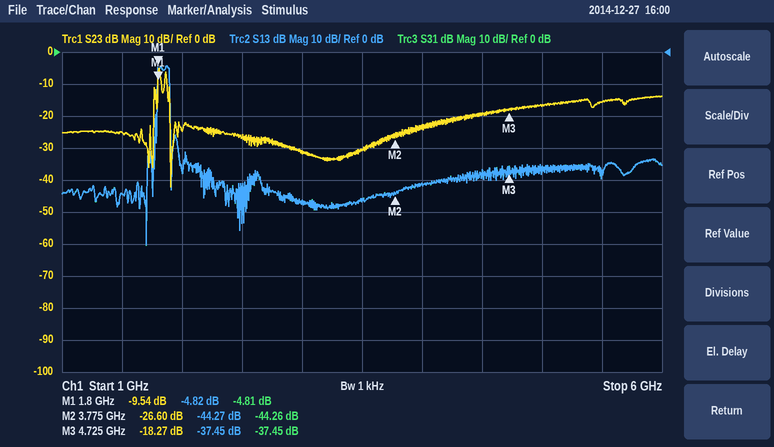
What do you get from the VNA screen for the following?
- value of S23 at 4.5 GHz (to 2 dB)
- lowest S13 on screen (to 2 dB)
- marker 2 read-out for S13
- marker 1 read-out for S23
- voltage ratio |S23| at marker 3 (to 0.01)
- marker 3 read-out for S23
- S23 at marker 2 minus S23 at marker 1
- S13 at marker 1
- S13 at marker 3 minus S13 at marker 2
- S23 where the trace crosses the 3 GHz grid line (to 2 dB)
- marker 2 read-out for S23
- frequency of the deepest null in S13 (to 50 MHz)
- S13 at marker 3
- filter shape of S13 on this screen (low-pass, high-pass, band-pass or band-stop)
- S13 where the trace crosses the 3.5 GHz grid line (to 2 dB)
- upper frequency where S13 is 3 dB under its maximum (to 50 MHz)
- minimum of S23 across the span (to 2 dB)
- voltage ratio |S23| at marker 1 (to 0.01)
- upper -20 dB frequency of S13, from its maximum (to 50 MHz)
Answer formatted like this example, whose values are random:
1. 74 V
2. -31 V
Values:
1. -20 dB
2. -60 dB
3. -44.27 dB
4. -9.54 dB
5. 0.12
6. -18.27 dB
7. -17.06 dB
8. -4.82 dB
9. 6.82 dB
10. -32 dB
11. -26.60 dB
12. 1.70 GHz
13. -37.45 dB
14. band-pass
15. -46 dB
16. 1.90 GHz
17. -42 dB
18. 0.33
19. 1.90 GHz
